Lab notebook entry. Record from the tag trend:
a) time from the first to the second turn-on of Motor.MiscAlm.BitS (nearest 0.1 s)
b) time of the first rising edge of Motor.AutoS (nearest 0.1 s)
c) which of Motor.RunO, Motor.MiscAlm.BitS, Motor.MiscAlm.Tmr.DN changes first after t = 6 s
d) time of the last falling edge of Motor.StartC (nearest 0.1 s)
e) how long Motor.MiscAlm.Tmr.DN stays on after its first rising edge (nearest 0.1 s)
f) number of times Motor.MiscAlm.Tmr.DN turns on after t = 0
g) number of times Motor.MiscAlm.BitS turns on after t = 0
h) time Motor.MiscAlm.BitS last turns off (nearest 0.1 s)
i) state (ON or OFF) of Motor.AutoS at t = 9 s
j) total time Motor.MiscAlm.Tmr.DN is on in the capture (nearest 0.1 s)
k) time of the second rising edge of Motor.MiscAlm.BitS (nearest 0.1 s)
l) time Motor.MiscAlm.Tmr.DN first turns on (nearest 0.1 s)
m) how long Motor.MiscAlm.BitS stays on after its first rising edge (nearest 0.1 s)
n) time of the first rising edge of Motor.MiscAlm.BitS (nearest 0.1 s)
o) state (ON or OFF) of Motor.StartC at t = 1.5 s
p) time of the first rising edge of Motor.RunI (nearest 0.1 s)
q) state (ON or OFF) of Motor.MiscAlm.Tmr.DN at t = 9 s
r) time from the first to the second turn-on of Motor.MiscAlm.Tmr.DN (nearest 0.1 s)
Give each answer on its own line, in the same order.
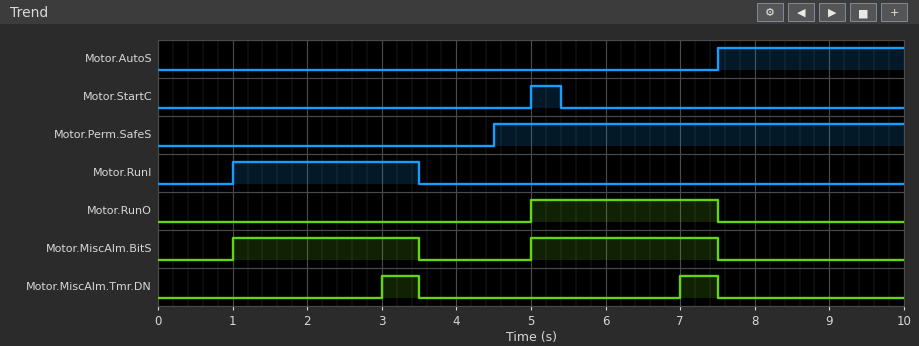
4.0 s
7.5 s
Motor.MiscAlm.Tmr.DN
5.4 s
0.5 s
2
2
7.5 s
ON
1.0 s
5.0 s
3.0 s
2.5 s
1.0 s
OFF
1.0 s
OFF
4.0 s
